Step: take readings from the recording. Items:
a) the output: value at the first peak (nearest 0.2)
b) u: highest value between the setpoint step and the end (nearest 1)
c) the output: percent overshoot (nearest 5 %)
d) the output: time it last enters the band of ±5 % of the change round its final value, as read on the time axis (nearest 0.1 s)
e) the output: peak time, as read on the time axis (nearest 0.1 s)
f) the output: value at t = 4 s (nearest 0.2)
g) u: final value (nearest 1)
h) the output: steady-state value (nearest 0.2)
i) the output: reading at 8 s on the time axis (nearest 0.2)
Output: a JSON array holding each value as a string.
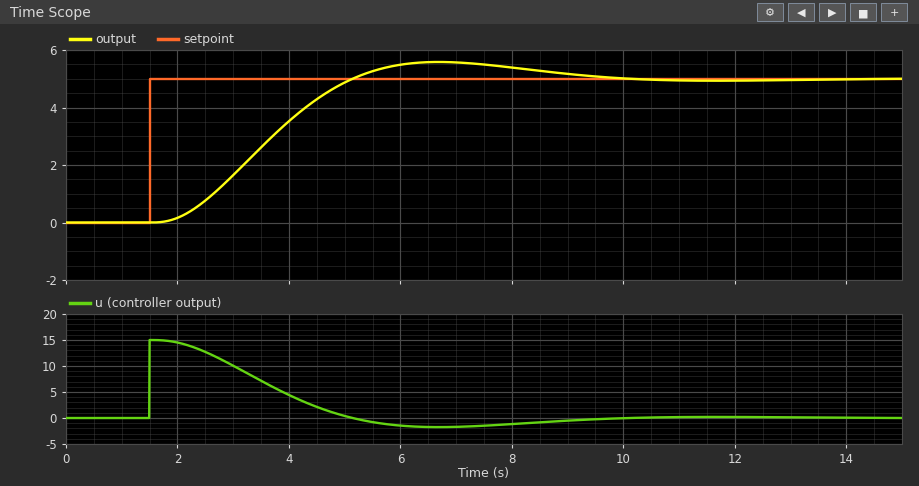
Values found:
["5.6", "15", "10 %", "8.6 s", "6.7 s", "3.6", "0", "5.0", "5.4"]
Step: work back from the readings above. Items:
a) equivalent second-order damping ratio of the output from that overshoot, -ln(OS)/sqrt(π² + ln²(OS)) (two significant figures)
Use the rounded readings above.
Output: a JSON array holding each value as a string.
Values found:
["0.59"]
